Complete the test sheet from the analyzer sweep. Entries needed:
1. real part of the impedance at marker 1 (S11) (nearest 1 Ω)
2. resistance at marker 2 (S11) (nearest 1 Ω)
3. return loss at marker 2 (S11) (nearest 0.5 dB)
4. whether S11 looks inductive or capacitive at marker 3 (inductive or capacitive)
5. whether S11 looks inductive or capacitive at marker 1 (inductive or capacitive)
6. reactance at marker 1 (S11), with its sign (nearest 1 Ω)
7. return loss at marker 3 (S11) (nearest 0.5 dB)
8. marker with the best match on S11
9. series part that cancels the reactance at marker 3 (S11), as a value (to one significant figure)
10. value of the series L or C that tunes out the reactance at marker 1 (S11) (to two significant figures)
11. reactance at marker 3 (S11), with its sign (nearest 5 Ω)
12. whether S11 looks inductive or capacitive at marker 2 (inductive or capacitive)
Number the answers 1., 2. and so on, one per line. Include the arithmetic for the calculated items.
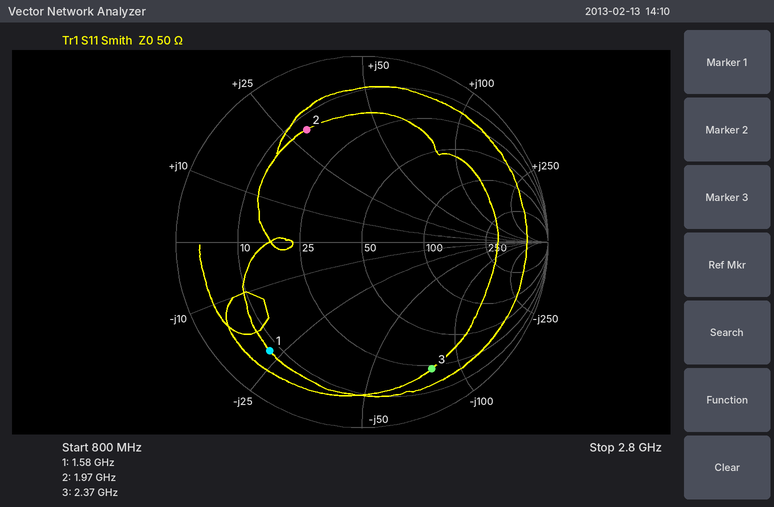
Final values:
1. 8 Ω
2. 13 Ω
3. 3.5 dB
4. capacitive
5. capacitive
6. -23 Ω
7. 2.0 dB
8. marker 2
9. L = 80 Ω/(2π × 2.37 GHz) ≈ 5 nH
10. L = 23 Ω/(2π × 1.58 GHz) ≈ 2.3 nH
11. -80 Ω
12. inductive
